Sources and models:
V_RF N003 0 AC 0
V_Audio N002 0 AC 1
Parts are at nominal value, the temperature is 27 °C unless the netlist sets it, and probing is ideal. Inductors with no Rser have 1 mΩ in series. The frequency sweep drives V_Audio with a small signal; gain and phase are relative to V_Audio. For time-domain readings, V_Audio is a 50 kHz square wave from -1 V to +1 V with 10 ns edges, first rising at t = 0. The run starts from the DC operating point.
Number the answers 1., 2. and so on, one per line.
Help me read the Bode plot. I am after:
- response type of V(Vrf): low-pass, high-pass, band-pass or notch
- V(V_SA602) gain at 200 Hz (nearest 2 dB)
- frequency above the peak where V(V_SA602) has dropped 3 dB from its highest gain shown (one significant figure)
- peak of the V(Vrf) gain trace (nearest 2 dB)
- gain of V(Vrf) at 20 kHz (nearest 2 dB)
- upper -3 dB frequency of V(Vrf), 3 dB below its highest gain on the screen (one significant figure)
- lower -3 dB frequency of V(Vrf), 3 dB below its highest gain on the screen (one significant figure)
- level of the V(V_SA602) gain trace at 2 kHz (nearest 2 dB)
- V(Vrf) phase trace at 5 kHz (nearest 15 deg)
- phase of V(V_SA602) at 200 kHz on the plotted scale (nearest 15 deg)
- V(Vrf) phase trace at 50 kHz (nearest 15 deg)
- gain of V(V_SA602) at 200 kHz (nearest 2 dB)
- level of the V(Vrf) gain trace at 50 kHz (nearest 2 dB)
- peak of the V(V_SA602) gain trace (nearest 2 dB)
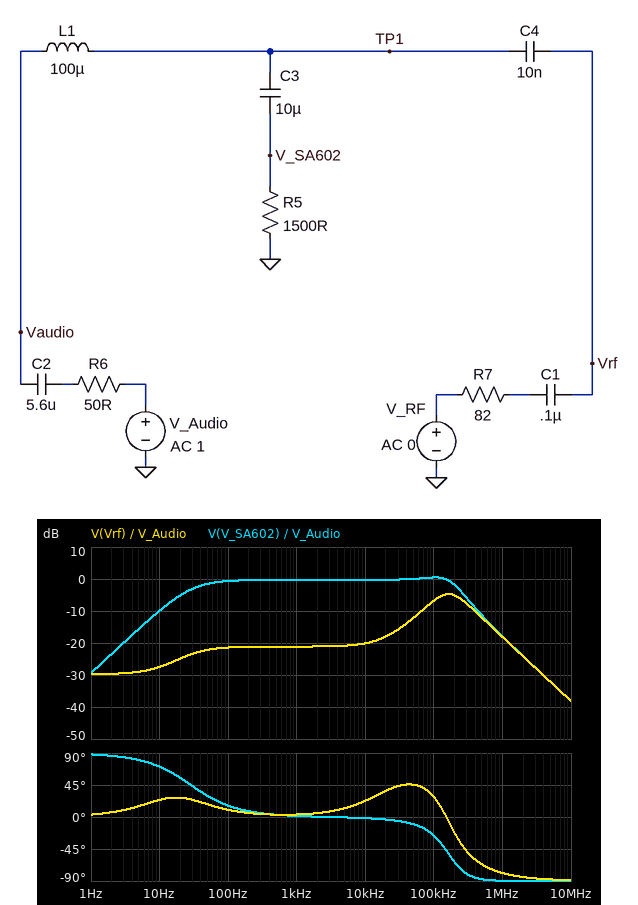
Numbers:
1. band-pass
2. 0 dB
3. 200 kHz
4. -4 dB
5. -18 dB
6. 300 kHz
7. 90 kHz
8. 0 dB
9. 15 deg
10. -60 deg
11. 45 deg
12. -2 dB
13. -12 dB
14. 0 dB
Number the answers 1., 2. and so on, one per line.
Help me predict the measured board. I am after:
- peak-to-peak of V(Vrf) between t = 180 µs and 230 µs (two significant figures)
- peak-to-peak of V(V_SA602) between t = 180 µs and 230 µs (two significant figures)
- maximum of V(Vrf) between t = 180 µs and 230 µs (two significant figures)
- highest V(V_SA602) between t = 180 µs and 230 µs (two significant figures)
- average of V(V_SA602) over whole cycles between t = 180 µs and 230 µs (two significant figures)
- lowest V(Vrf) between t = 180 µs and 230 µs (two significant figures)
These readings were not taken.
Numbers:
1. 1.4 V
2. 2.4 V
3. 790 mV
4. 2.1 V
5. 930 mV
6. -610 mV
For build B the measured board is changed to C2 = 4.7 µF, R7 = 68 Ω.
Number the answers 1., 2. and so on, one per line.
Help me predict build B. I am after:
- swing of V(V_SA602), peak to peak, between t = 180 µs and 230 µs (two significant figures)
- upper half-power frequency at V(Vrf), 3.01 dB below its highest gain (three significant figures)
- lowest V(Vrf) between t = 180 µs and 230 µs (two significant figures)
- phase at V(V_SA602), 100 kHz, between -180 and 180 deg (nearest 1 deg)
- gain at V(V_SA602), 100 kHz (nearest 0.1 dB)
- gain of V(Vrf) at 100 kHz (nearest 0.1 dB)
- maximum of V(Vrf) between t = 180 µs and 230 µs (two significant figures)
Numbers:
1. 2.5 V
2. 288 kHz
3. -540 mV
4. -27 deg
5. 0.8 dB
6. -7.8 dB
7. 710 mV
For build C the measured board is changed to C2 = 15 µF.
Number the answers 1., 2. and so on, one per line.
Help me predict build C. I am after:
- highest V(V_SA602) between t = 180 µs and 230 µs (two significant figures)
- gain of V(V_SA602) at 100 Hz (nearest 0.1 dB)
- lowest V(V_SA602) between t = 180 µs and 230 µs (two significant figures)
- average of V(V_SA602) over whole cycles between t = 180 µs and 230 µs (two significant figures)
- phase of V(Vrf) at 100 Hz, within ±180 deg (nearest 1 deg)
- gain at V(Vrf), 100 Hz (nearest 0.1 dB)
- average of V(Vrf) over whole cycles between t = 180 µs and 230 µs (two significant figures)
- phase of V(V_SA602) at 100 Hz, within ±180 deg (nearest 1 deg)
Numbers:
1. 2.1 V
2. -0.4 dB
3. -240 mV
4. 950 mV
5. 4 deg
6. -21.2 dB
7. 87 mV
8. 10 deg
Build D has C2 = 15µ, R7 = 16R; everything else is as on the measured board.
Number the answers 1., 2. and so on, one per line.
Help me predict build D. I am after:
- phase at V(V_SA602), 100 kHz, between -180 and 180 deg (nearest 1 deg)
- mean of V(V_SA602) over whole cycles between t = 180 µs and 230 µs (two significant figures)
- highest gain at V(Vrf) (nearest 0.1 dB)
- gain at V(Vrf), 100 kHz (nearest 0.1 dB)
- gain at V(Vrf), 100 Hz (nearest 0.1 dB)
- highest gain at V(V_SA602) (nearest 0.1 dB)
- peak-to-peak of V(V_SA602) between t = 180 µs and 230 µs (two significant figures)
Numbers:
1. -27 deg
2. 950 mV
3. -12.0 dB
4. -15.8 dB
5. -21.2 dB
6. 3.6 dB
7. 3.2 V
